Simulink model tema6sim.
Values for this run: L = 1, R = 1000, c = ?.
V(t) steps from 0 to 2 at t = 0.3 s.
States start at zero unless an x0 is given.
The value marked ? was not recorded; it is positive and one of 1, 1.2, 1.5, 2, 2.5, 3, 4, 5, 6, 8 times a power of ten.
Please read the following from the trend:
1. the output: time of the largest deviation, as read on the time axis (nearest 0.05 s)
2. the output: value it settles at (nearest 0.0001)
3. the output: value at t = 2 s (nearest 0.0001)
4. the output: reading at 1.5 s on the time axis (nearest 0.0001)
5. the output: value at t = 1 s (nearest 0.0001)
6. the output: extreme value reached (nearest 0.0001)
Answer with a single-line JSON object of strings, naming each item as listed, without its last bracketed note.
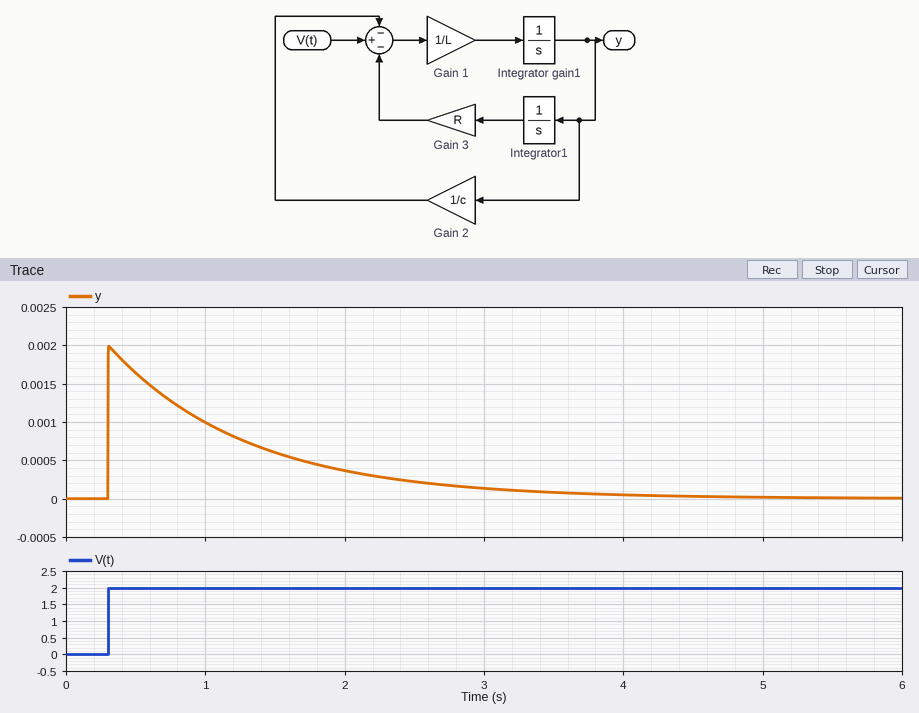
{"the output: time of the largest deviation, as read on the time axis": "0.30 s", "the output: value it settles at": "0.0000", "the output: value at t = 2 s": "0.0004", "the output: reading at 1.5 s on the time axis": "0.0006", "the output: value at t = 1 s": "0.0010", "the output: extreme value reached": "0.0020"}
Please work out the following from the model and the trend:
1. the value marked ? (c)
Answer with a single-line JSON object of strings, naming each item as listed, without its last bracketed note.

{"the value marked ?": "0.001"}
